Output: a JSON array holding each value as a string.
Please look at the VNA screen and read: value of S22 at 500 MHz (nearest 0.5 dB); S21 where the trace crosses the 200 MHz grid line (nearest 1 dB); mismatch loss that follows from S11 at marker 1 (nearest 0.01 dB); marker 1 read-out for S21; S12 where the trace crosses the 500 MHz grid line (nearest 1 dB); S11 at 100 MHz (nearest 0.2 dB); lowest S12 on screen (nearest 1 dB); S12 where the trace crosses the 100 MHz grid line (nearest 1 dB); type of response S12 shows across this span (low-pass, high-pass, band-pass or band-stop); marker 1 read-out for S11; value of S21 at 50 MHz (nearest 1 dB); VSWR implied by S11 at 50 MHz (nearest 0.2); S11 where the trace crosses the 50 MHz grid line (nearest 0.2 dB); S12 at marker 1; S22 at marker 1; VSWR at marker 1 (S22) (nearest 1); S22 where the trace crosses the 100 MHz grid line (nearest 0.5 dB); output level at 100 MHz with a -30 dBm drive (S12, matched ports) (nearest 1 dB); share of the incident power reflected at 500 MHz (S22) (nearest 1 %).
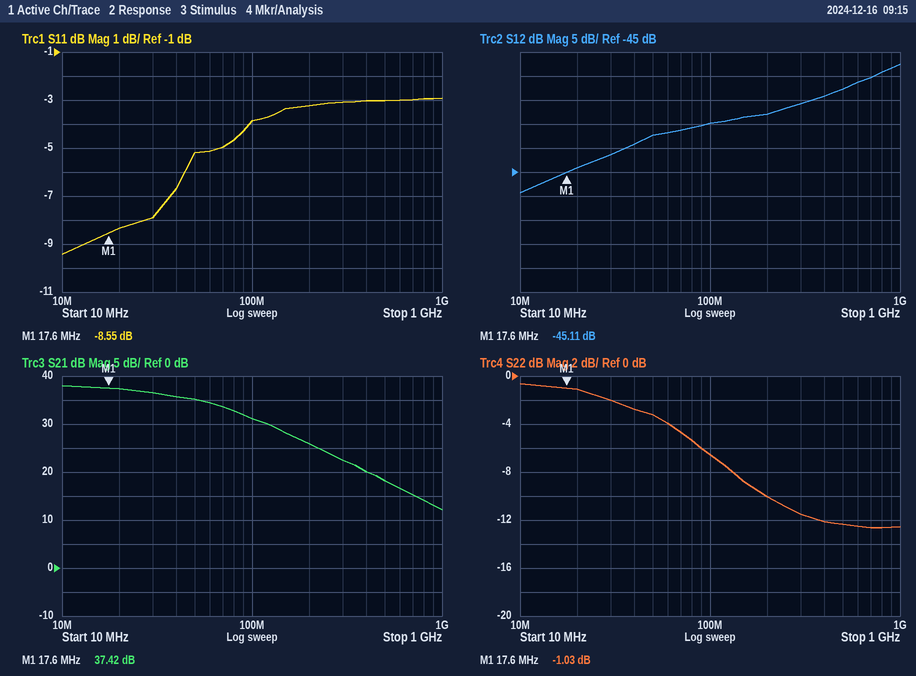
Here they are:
["-12.5 dB", "26 dB", "0.65 dB", "37.42 dB", "-28 dB", "-3.8 dB", "-49 dB", "-35 dB", "high-pass", "-8.55 dB", "35 dB", "3.4", "-5.2 dB", "-45.11 dB", "-1.03 dB", "17", "-6.5 dB", "-65 dBm", "6 %"]
